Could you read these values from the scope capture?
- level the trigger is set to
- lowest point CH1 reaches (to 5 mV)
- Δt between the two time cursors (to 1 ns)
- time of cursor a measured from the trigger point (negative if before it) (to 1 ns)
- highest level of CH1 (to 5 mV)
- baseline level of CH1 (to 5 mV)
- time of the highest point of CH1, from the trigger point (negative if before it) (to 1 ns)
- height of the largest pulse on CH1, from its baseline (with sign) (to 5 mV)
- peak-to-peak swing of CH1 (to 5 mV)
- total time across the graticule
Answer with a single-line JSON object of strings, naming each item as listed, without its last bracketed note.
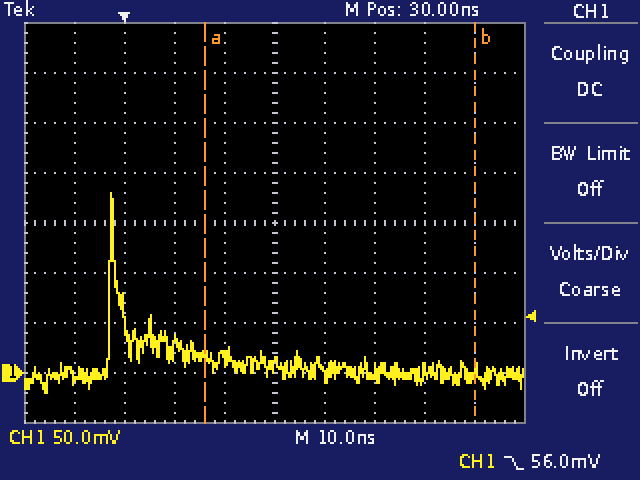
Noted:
{"level the trigger is set to": "56.0 mV", "lowest point CH1 reaches": "-20 mV", "Δt between the two time cursors": "54 ns", "time of cursor a measured from the trigger point (negative if before it)": "+16 ns", "highest level of CH1": "180 mV", "baseline level of CH1": "0 mV", "time of the highest point of CH1, from the trigger point (negative if before it)": "-3 ns", "height of the largest pulse on CH1, from its baseline (with sign)": "+180 mV", "peak-to-peak swing of CH1": "200 mV", "total time across the graticule": "100 ns"}
